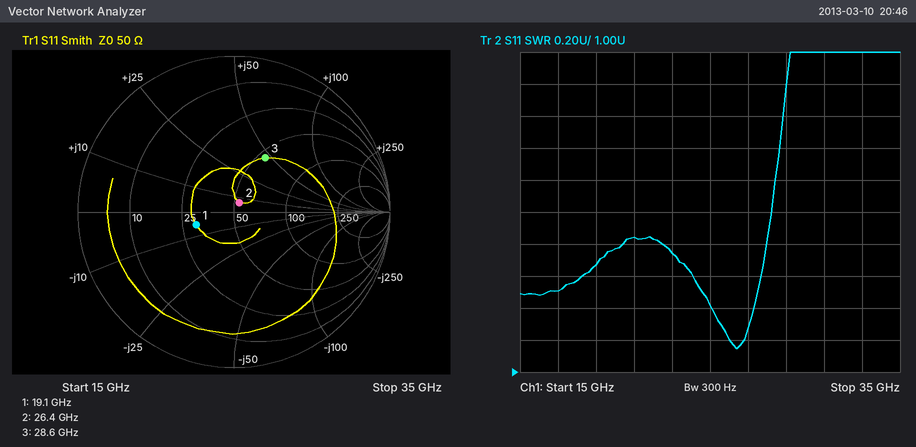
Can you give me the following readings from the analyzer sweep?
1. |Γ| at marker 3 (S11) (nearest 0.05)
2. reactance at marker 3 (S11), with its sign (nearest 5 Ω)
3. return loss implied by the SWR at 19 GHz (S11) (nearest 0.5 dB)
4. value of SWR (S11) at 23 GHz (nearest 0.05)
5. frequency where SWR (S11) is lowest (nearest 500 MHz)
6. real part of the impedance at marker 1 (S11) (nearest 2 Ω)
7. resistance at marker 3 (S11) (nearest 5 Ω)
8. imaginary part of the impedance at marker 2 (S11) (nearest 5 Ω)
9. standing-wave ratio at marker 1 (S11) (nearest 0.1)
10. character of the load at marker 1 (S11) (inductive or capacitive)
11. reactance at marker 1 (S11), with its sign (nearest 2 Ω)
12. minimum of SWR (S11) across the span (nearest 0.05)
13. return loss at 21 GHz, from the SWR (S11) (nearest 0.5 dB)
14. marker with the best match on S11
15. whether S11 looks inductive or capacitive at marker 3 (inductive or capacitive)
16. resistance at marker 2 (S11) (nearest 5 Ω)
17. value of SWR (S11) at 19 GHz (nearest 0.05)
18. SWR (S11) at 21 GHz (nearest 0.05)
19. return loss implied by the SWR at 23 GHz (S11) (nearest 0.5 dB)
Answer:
0.40
+45 Ω
12.0 dB
1.75
26.5 GHz
30 Ω
55 Ω
+5 Ω
1.7
capacitive
-6 Ω
1.15
10.5 dB
marker 2
inductive
55 Ω
1.65
1.85
11.5 dB
